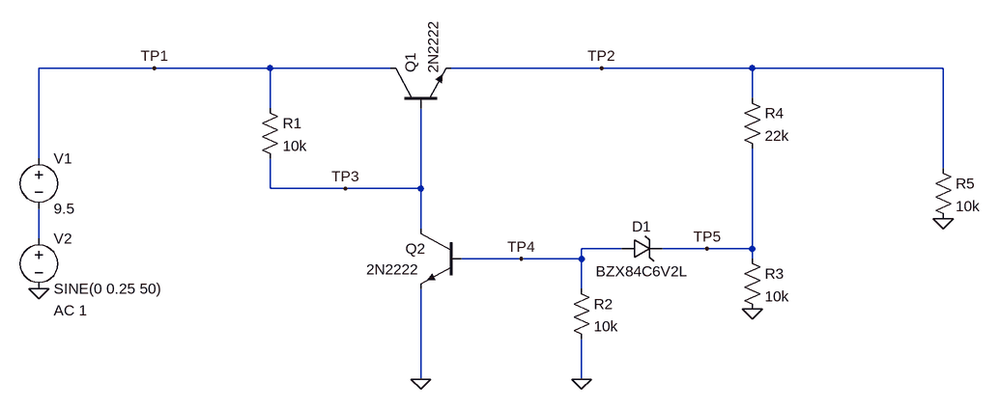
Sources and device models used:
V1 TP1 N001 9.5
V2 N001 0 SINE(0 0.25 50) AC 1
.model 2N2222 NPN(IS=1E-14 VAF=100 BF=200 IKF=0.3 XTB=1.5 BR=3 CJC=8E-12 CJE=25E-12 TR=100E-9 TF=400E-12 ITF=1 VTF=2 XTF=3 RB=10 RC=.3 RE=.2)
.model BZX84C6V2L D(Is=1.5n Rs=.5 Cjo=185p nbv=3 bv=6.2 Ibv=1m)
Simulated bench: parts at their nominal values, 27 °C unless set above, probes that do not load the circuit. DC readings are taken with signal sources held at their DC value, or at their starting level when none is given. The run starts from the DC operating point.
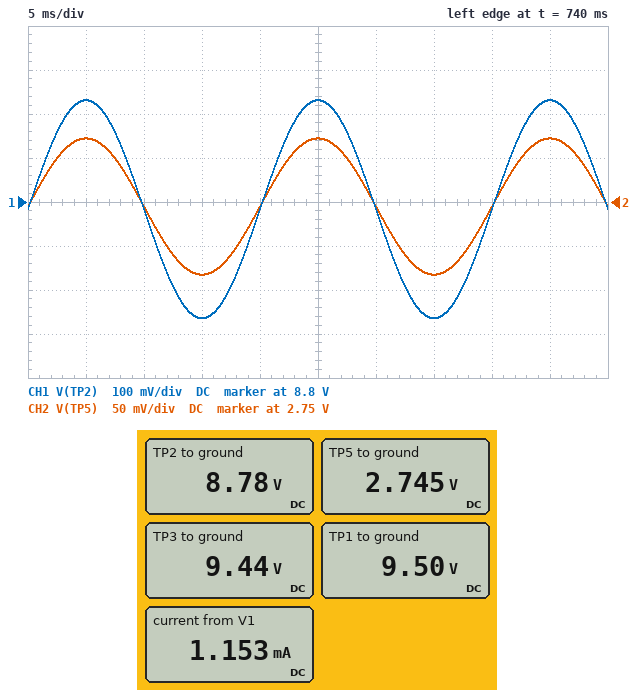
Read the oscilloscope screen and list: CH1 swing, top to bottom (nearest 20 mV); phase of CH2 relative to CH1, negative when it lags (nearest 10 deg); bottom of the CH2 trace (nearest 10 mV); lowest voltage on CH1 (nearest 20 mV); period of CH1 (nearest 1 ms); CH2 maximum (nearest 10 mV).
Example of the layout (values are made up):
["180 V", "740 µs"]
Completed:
["500 mV", "0 deg", "2.67 V", "8.54 V", "20 ms", "2.82 V"]
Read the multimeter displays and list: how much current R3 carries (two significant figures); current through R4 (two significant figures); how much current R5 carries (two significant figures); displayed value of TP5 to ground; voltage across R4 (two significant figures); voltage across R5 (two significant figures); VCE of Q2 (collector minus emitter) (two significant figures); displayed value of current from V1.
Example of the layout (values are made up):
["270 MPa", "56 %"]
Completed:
["270 µA", "270 µA", "880 µA", "2.745 V", "6.0 V", "8.8 V", "9.4 V", "1.153 mA"]
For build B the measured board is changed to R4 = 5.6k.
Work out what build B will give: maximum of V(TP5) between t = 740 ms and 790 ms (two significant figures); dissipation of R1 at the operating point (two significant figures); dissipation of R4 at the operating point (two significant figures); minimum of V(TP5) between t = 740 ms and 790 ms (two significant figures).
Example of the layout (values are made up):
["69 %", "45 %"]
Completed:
["5.8 V", "520 nW", "1.8 mW", "5.5 V"]
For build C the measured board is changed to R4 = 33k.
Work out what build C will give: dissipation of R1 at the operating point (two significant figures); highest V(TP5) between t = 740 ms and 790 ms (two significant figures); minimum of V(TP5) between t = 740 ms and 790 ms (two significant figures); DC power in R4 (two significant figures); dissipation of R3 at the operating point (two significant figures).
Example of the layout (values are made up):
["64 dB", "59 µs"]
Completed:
["290 nW", "2.1 V", "2.0 V", "1.4 mW", "420 µW"]
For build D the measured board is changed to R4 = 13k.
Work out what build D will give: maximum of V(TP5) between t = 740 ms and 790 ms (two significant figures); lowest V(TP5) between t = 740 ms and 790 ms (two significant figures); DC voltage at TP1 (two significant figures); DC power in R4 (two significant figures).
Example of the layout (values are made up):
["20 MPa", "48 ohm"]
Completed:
["3.9 V", "3.7 V", "9.5 V", "1.9 mW"]
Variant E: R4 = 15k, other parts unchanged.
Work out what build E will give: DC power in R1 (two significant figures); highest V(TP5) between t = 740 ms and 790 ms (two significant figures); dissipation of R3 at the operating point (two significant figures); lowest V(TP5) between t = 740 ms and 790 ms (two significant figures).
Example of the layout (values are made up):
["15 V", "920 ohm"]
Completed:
["380 nW", "3.6 V", "1.2 mW", "3.4 V"]
